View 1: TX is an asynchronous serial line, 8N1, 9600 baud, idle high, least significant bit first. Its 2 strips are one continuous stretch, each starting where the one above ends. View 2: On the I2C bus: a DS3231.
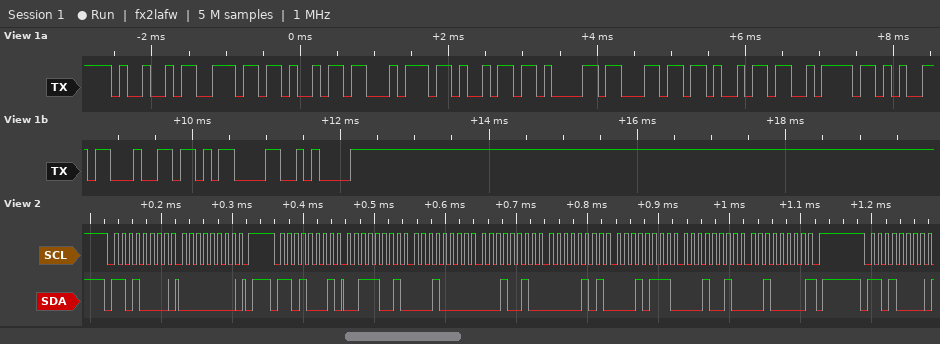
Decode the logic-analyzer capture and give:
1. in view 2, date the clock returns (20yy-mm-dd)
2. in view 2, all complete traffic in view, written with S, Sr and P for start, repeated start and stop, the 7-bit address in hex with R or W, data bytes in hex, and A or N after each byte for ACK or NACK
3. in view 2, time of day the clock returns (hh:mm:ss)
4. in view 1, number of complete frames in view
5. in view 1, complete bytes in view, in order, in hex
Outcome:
2020-12-17
S 68W A 00 A P S 68R A 39 A 10 A 12 A 05 A 17 A 12 A 20 N P S 68W A
12:10:39
13
0x49 0x6E 0x69 0x74 0x69 0x61 0x6C 0x69 0x7A 0x65 0x64 0x0D 0x0A
